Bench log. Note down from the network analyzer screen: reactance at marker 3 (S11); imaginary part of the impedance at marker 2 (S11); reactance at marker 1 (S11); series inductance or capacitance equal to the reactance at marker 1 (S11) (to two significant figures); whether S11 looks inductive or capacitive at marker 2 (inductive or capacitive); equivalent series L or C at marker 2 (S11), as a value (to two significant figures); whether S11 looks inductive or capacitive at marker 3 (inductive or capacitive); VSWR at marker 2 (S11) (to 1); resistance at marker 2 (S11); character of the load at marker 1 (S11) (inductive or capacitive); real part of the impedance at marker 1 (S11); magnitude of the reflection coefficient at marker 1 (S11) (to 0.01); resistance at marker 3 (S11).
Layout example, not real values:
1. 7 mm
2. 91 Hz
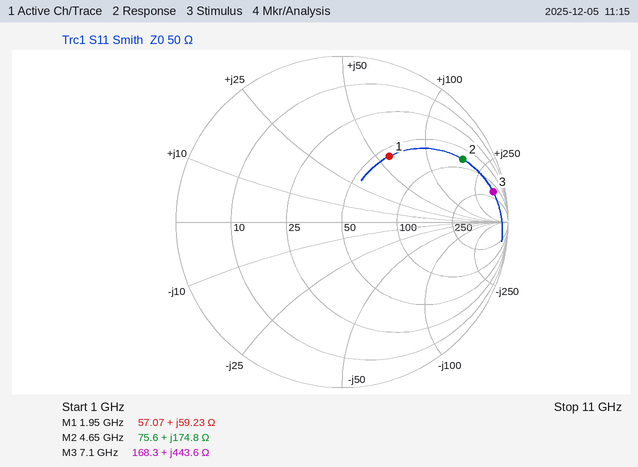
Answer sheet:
1. +443.6 Ω
2. +174.8 Ω
3. +59.23 Ω
4. 4.8 nH
5. inductive
6. 6.0 nH
7. inductive
8. 10
9. 75.6 Ω
10. inductive
11. 57.07 Ω
12. 0.49
13. 168.3 Ω
